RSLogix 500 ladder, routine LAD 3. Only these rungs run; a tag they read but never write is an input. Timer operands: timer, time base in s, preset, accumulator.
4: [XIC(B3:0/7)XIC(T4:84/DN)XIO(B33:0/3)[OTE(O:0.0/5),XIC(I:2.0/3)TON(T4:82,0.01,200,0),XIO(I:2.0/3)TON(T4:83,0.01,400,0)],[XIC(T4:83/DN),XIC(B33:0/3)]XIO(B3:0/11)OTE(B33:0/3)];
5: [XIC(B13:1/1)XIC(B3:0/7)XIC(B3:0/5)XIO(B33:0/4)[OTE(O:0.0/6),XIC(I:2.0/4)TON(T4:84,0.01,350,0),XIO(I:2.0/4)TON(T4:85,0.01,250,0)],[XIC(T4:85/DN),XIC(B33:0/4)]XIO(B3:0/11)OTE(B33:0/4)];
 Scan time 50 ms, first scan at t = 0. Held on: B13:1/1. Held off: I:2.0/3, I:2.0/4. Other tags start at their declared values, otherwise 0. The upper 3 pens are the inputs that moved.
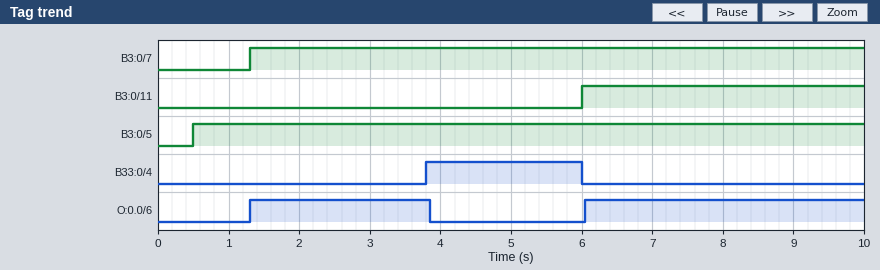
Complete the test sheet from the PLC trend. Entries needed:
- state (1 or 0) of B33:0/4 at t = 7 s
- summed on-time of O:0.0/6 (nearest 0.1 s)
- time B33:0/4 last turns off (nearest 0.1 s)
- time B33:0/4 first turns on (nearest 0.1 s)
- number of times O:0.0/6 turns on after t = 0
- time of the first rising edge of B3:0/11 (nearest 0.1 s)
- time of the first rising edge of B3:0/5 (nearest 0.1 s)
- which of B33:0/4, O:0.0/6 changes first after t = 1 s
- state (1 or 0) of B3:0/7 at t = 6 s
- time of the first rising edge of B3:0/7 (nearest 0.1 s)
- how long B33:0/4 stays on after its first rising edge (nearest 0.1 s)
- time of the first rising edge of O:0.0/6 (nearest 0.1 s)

0
6.5 s
6.0 s
3.8 s
2
6.0 s
0.5 s
O:0.0/6
1
1.3 s
2.2 s
1.3 s
